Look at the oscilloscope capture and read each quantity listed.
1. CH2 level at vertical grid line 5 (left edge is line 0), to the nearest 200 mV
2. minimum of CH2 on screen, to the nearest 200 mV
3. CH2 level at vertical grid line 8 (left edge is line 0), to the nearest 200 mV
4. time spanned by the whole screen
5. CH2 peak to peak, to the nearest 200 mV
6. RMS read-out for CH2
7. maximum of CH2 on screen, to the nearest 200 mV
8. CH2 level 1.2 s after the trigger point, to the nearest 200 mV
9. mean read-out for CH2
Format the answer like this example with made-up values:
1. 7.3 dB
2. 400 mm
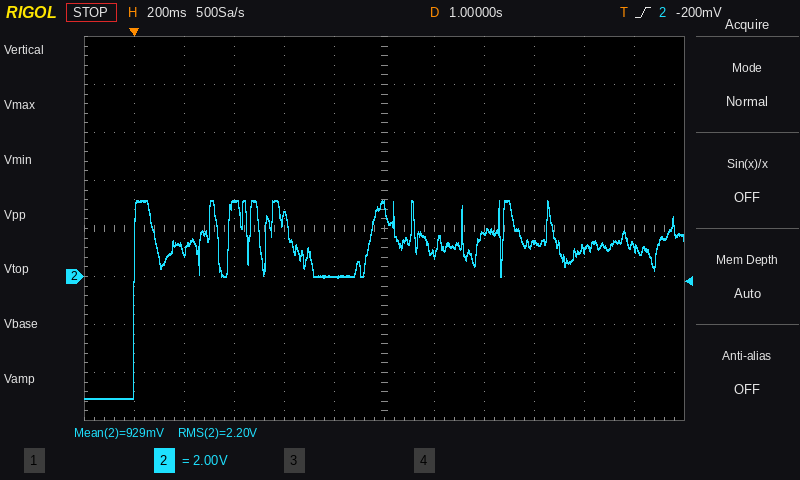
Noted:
1. 0.0 V
2. -5.0 V
3. 1.8 V
4. 2.4 s
5. 8.2 V
6. 2.20 V
7. 3.2 V
8. 1.0 V
9. 929 mV
